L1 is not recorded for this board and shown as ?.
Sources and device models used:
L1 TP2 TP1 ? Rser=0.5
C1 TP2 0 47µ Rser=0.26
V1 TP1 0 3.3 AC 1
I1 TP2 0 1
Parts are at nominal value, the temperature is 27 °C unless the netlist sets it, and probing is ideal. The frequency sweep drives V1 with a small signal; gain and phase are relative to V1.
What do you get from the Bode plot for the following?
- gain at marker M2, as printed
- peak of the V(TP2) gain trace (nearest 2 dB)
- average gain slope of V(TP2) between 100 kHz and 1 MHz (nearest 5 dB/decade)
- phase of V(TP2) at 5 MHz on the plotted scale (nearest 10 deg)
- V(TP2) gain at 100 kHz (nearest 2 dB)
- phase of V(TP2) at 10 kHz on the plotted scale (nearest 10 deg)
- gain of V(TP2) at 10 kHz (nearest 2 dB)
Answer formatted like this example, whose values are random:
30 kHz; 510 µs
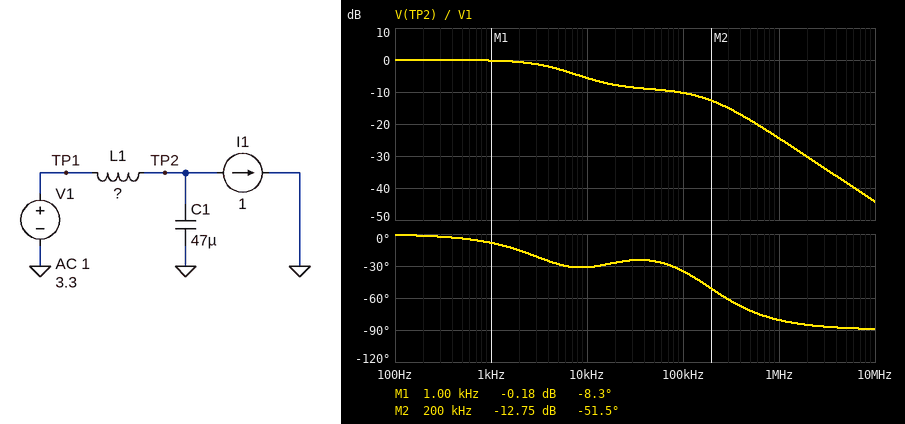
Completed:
-12.75 dB; 0 dB; -15 dB/decade; -90 deg; -10 dB; -30 deg; -6 dB
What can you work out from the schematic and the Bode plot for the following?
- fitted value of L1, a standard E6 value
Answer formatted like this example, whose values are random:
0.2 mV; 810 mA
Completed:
680 nH
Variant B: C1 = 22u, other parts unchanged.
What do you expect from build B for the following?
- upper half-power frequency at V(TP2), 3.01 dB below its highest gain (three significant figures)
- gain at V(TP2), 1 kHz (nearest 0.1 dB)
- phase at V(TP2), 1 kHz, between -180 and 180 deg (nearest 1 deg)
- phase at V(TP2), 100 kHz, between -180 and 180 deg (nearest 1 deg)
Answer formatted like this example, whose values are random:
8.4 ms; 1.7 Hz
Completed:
11.7 kHz; 0 dB; -4 deg; -41 deg
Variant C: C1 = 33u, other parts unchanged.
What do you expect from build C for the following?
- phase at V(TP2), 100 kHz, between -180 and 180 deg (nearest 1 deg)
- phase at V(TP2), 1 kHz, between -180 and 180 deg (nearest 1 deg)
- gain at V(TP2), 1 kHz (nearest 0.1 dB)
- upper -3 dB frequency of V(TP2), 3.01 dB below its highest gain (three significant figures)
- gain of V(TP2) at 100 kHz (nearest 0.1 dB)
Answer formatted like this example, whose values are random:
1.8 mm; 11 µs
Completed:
-37 deg; -6 deg; -0.1 dB; 7.60 kHz; -10.1 dB
